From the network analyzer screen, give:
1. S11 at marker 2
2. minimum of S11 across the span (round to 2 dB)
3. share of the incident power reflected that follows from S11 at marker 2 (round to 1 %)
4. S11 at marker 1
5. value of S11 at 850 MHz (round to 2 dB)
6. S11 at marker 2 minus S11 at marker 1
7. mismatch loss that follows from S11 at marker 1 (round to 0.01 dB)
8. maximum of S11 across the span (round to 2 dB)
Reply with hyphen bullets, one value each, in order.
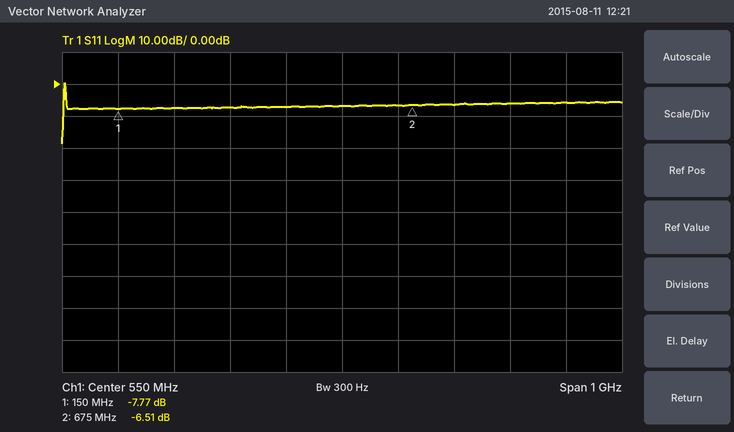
- -6.51 dB
- -18 dB
- 22 %
- -7.77 dB
- -6 dB
- 1.26 dB
- 0.79 dB
- 0 dB
